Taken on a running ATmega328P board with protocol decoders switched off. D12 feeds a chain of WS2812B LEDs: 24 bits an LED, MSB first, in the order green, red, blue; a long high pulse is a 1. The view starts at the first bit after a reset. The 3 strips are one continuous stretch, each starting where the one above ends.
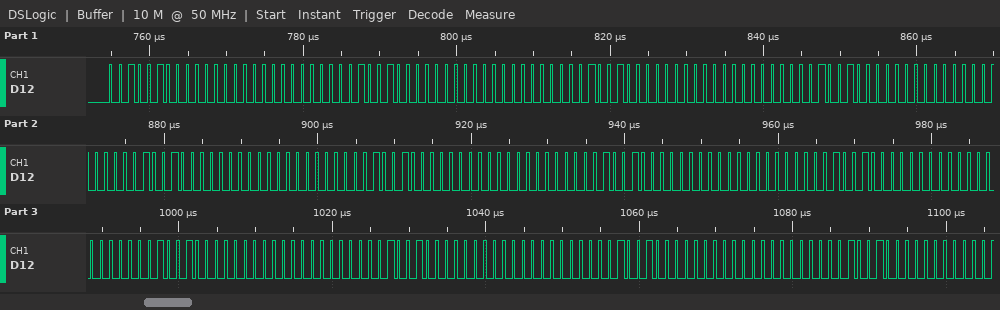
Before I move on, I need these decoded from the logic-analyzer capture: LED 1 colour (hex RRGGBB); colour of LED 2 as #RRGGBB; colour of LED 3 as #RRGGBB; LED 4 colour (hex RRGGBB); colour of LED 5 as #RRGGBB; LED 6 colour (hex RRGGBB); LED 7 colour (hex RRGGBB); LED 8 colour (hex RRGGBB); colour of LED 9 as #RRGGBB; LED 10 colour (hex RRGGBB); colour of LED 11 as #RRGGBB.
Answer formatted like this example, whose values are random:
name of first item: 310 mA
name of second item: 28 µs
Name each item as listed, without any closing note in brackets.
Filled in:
LED 1 colour: #002400
colour of LED 2 as #RRGGBB: #002400
colour of LED 3 as #RRGGBB: #002400
LED 4 colour: #002400
colour of LED 5 as #RRGGBB: #002400
LED 6 colour: #002400
LED 7 colour: #002400
LED 8 colour: #002400
colour of LED 9 as #RRGGBB: #002400
LED 10 colour: #002400
colour of LED 11 as #RRGGBB: #002400
